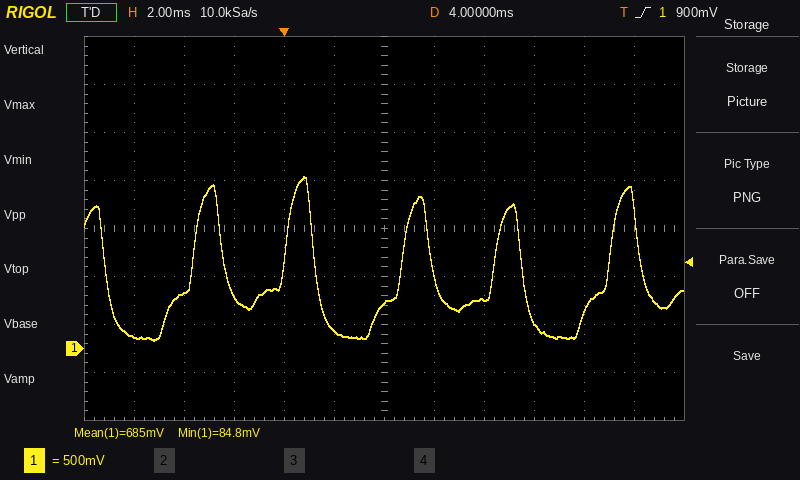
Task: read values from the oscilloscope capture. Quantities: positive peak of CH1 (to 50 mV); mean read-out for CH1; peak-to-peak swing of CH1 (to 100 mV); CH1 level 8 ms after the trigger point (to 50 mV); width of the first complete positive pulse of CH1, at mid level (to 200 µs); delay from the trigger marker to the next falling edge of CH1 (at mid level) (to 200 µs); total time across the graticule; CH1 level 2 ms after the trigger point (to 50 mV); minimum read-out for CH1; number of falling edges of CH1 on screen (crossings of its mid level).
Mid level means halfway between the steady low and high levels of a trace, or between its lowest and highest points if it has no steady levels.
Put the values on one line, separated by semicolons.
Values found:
1.80 V; 685 mV; 1.70 V; 500 mV; 1.2 ms; 1.2 ms; 24 ms; 200 mV; 84.8 mV; 6
